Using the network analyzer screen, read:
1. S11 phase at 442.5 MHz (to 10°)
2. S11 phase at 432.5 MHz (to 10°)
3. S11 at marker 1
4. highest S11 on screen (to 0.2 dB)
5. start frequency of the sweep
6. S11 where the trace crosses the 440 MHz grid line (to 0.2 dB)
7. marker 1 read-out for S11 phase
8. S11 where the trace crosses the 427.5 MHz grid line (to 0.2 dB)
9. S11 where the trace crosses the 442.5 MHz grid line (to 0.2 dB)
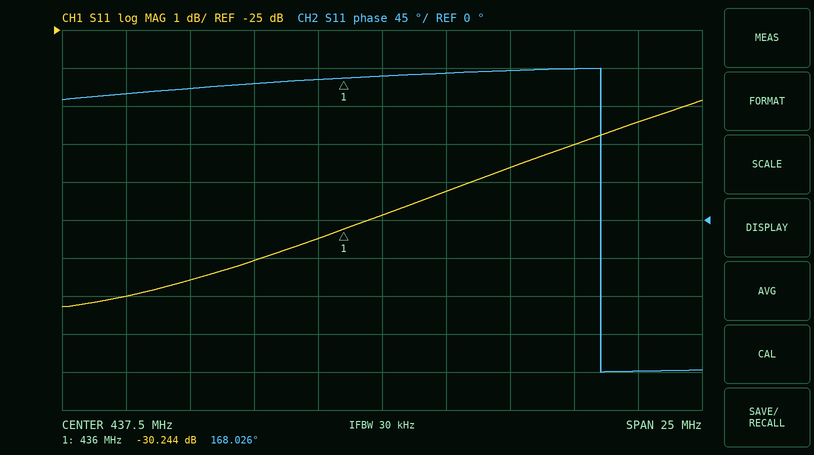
180°
160°
-30.244 dB
-26.8 dB
425 MHz
-29.2 dB
168.026°
-32.0 dB
-28.6 dB
